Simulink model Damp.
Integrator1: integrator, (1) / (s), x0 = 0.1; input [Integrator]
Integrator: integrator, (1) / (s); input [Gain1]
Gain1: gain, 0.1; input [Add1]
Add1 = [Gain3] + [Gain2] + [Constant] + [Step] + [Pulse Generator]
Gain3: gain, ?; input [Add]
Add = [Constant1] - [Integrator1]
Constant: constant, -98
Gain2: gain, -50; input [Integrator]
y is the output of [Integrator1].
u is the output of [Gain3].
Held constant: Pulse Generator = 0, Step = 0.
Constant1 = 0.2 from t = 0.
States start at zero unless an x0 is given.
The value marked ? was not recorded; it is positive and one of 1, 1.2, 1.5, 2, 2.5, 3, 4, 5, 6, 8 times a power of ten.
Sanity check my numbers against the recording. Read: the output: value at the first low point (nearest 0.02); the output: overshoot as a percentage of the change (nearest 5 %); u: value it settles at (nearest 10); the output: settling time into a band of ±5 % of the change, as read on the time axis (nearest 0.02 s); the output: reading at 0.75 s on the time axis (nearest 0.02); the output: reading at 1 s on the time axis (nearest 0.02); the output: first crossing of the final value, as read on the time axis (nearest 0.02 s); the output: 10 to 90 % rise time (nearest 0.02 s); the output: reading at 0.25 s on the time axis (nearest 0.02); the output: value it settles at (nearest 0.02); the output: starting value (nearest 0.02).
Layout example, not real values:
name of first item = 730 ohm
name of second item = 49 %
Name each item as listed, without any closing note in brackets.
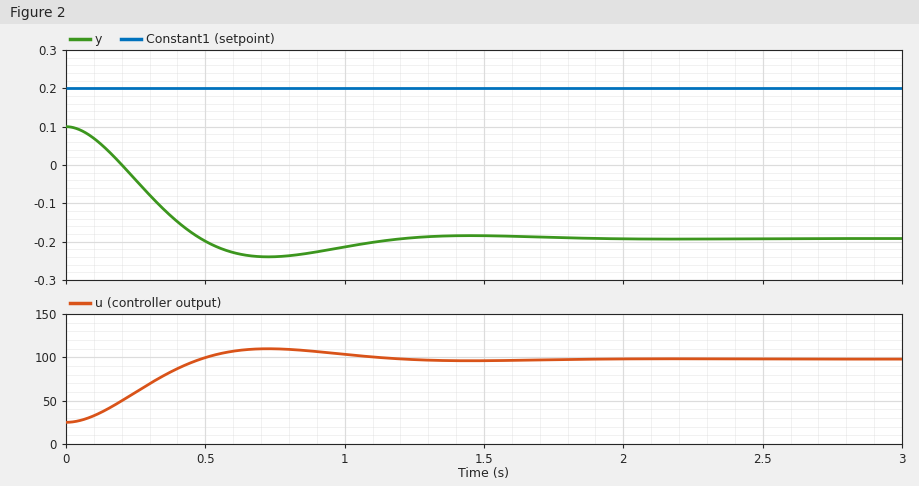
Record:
the output: value at the first low point = -0.24
the output: overshoot as a percentage of the change = 15 %
u: value it settles at = 100
the output: settling time into a band of ±5 % of the change, as read on the time axis = 1.06 s
the output: reading at 0.75 s on the time axis = -0.24
the output: reading at 1 s on the time axis = -0.22
the output: first crossing of the final value, as read on the time axis = 0.48 s
the output: 10 to 90 % rise time = 0.32 s
the output: reading at 0.25 s on the time axis = -0.04
the output: value it settles at = -0.20
the output: starting value = 0.10
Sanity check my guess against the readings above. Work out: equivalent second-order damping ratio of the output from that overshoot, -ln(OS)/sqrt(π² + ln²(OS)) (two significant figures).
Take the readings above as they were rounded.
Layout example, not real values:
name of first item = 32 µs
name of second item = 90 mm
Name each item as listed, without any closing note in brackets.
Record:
equivalent second-order damping ratio of the output from that overshoot, -ln(OS)/sqrt(π² + ln²(OS)) = 0.52
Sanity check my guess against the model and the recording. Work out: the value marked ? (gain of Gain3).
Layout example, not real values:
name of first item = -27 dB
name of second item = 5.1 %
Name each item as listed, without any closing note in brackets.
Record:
the value marked ? = 250
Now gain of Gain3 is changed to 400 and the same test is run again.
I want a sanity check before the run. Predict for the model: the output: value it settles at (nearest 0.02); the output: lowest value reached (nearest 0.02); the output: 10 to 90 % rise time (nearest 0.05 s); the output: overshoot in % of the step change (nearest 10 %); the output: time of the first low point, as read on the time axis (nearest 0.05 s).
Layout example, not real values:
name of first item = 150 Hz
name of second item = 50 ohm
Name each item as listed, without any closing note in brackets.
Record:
the output: value it settles at = -0.04
the output: lowest value reached = -0.08
the output: 10 to 90 % rise time = 0.25 s
the output: overshoot in % of the step change = 30 %
the output: time of the first low point, as read on the time axis = 0.55 s
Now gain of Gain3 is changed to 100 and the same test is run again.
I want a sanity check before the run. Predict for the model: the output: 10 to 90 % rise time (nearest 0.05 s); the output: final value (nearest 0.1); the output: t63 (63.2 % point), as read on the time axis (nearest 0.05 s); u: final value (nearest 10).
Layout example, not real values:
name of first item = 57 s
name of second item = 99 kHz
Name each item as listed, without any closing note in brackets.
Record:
the output: 10 to 90 % rise time = 0.75 s
the output: final value = -0.8
the output: t63 (63.2 % point), as read on the time axis = 0.60 s
u: final value = 100
